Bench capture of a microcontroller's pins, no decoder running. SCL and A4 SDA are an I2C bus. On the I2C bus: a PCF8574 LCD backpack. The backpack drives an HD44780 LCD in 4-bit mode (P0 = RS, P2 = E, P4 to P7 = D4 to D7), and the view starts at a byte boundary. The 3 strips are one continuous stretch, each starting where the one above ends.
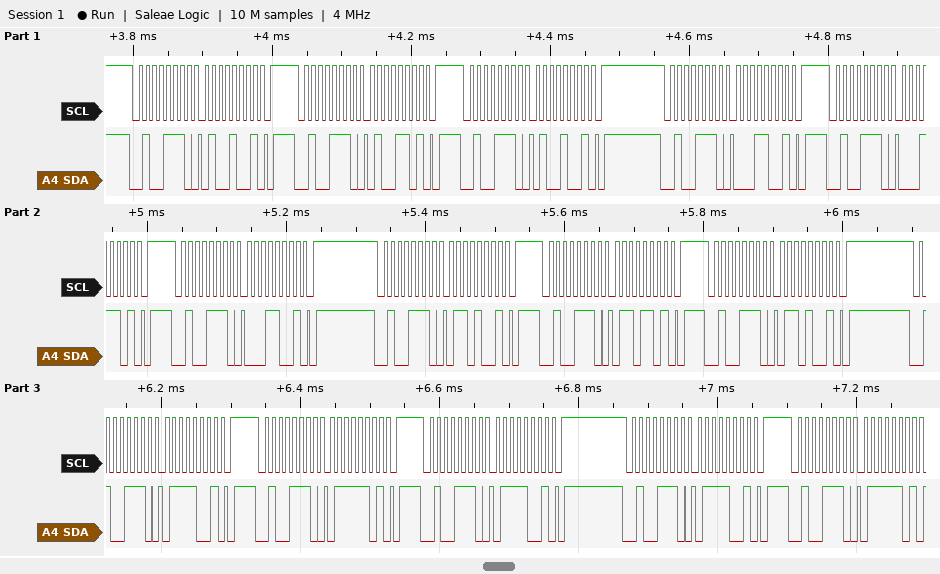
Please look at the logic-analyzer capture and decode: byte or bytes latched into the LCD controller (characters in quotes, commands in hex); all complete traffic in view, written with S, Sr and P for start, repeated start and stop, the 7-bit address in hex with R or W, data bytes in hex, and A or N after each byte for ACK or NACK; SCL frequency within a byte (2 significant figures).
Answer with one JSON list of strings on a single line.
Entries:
["'A' 'g'", "S 27W A 49 A P S 27W A 4D A P S 27W A 49 A P S 27W A 19 A P S 27W A 1D A P S 27W A 19 A P S 27W A 69 A P S 27W A 6D A P S 27W A 69 A P S 27W A 79 A P S 27W A 7D A P S 27W A 79 A P S 27W A 79 A P S 27W A 7D A", "100 kHz"]
